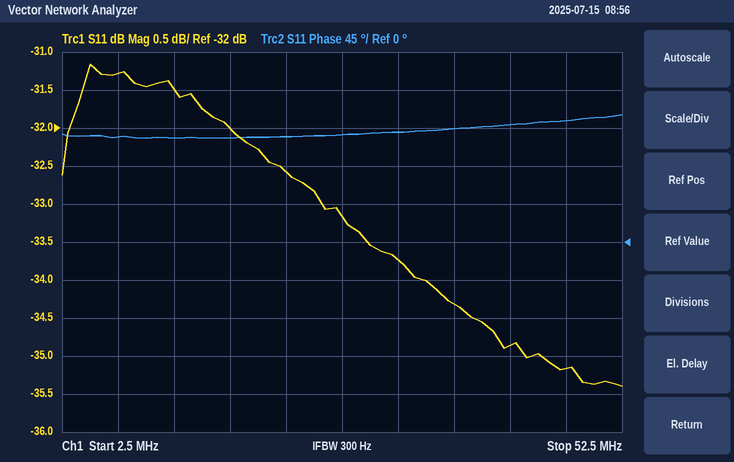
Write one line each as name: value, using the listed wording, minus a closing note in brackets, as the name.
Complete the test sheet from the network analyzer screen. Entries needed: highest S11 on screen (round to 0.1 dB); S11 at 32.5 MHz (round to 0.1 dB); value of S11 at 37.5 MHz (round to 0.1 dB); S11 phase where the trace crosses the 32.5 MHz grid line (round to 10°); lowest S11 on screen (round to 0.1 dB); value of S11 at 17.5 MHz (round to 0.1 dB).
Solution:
highest S11 on screen: -31.2 dB
S11 at 32.5 MHz: -33.7 dB
value of S11 at 37.5 MHz: -34.3 dB
S11 phase where the trace crosses the 32.5 MHz grid line: 130°
lowest S11 on screen: -35.4 dB
value of S11 at 17.5 MHz: -32.0 dB
